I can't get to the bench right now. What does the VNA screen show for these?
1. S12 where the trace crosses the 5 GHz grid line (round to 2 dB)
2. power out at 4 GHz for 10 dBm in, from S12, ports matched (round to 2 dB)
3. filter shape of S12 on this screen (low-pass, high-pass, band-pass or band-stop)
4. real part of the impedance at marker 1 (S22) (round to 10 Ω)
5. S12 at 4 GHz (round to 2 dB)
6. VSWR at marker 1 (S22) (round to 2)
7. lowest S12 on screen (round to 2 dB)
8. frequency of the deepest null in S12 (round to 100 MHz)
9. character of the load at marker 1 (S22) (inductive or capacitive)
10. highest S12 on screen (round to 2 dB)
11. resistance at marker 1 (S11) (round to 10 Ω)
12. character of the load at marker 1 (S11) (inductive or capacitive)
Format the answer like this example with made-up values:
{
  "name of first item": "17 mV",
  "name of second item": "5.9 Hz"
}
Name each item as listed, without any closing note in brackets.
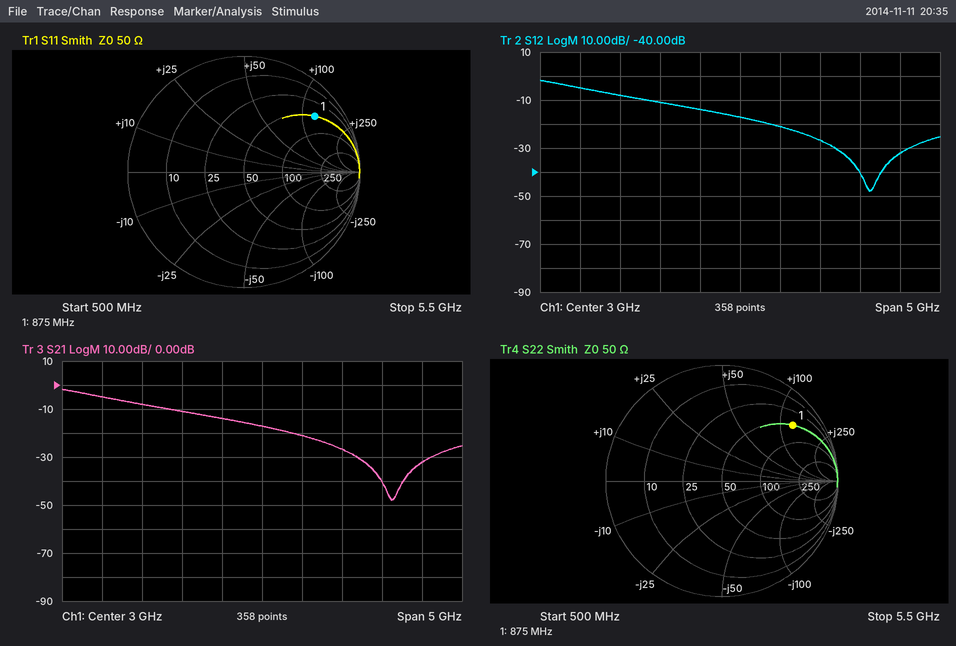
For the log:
{
  "S12 where the trace crosses the 5 GHz grid line": "-32 dB",
  "power out at 4 GHz for 10 dBm in, from S12, ports matched": "-16 dBm",
  "filter shape of S12 on this screen": "low-pass",
  "real part of the impedance at marker 1 (S22)": "50 Ω",
  "S12 at 4 GHz": "-26 dB",
  "VSWR at marker 1 (S22)": "8",
  "lowest S12 on screen": "-48 dB",
  "frequency of the deepest null in S12": "4.6 GHz",
  "character of the load at marker 1 (S22)": "inductive",
  "highest S12 on screen": "-2 dB",
  "resistance at marker 1 (S11)": "50 Ω",
  "character of the load at marker 1 (S11)": "inductive"
}
